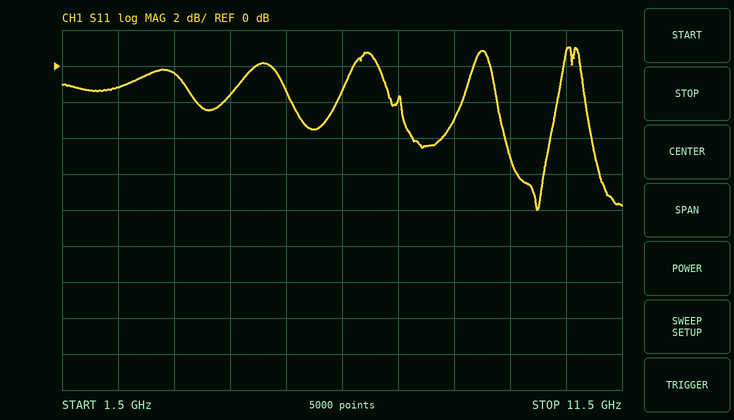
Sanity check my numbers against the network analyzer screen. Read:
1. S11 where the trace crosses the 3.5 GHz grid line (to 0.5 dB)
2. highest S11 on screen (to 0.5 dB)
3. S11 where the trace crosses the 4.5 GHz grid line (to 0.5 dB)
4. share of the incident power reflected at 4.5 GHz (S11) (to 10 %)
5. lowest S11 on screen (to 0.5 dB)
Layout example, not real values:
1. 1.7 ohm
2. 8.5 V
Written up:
1. -0.5 dB
2. 1.0 dB
3. -1.5 dB
4. 70 %
5. -8.0 dB
